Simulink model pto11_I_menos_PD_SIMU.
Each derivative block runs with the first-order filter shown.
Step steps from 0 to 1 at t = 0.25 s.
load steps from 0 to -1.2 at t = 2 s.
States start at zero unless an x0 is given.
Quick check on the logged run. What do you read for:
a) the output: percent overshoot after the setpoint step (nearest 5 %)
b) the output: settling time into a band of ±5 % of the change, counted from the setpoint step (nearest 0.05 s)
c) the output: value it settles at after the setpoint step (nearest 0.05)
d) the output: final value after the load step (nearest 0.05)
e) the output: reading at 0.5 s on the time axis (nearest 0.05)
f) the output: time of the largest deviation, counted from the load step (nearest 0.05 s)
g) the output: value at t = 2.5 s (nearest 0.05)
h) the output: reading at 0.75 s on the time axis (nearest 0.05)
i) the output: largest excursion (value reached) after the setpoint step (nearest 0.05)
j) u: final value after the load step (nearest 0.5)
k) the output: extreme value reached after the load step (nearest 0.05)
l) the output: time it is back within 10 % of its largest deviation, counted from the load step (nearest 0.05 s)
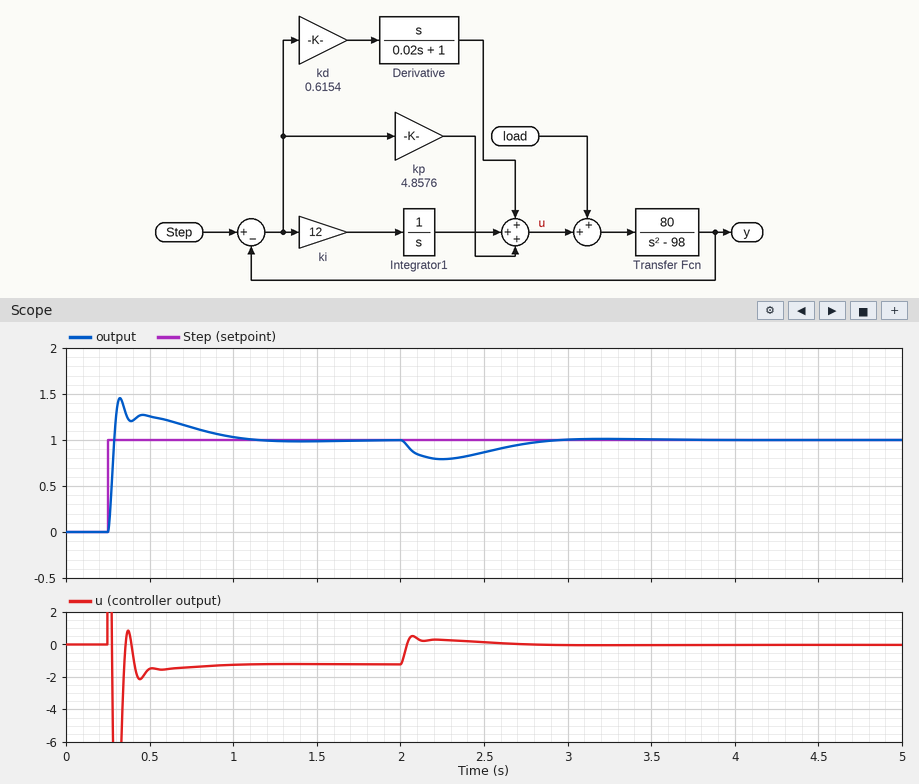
45 %
0.70 s
1.00
1.00
1.25
0.25 s
0.85
1.15
1.45
0.0
0.80
0.85 s
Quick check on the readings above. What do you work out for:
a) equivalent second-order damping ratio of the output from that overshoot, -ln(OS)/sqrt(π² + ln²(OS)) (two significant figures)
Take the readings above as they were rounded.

0.25
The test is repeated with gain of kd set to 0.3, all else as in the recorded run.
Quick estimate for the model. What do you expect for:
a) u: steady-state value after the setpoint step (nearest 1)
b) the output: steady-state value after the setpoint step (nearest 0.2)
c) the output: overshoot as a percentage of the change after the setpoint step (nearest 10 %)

-1
1.0
70 %
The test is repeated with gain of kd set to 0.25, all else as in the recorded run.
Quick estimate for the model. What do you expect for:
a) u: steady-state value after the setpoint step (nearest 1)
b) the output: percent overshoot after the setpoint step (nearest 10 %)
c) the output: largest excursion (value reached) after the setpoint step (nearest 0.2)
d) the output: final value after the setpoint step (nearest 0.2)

-1
80 %
1.8
1.0
